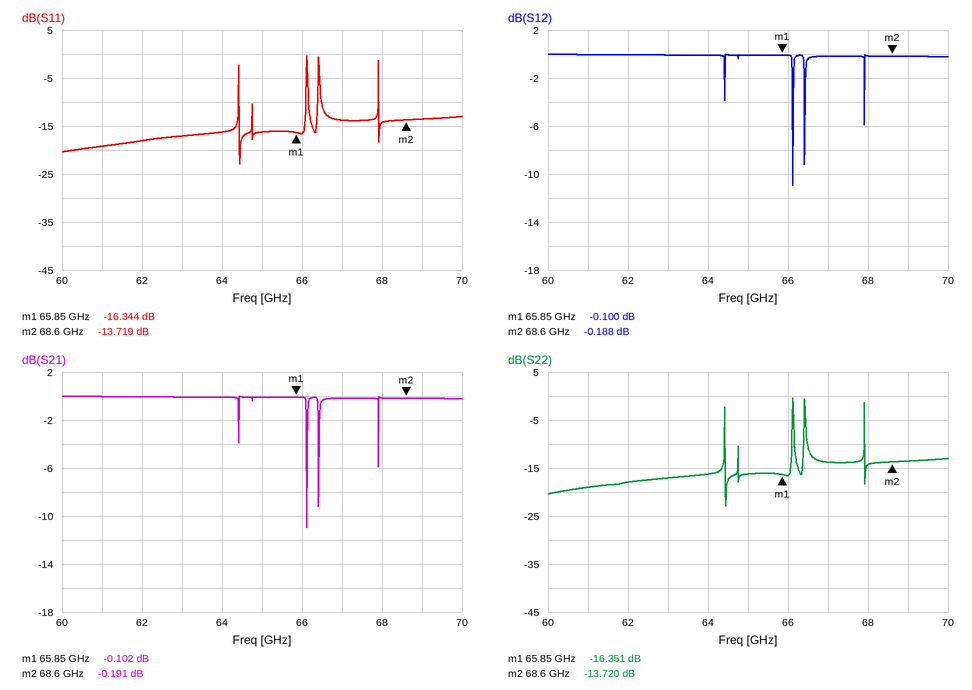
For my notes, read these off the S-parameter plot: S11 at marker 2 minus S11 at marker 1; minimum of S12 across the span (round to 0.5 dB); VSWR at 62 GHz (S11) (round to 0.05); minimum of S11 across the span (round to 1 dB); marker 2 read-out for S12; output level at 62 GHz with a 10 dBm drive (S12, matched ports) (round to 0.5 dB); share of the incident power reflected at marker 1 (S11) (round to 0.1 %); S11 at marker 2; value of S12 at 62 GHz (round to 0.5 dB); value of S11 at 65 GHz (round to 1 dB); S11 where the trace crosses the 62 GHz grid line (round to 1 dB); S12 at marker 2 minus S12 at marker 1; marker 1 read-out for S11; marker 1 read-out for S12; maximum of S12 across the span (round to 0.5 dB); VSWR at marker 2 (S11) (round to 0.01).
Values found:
2.625 dB
-11.0 dB
1.30
-23 dB
-0.188 dB
10.0 dBm
2.3 %
-13.719 dB
0.0 dB
-16 dB
-18 dB
-0.088 dB
-16.344 dB
-0.100 dB
0.0 dB
1.52
